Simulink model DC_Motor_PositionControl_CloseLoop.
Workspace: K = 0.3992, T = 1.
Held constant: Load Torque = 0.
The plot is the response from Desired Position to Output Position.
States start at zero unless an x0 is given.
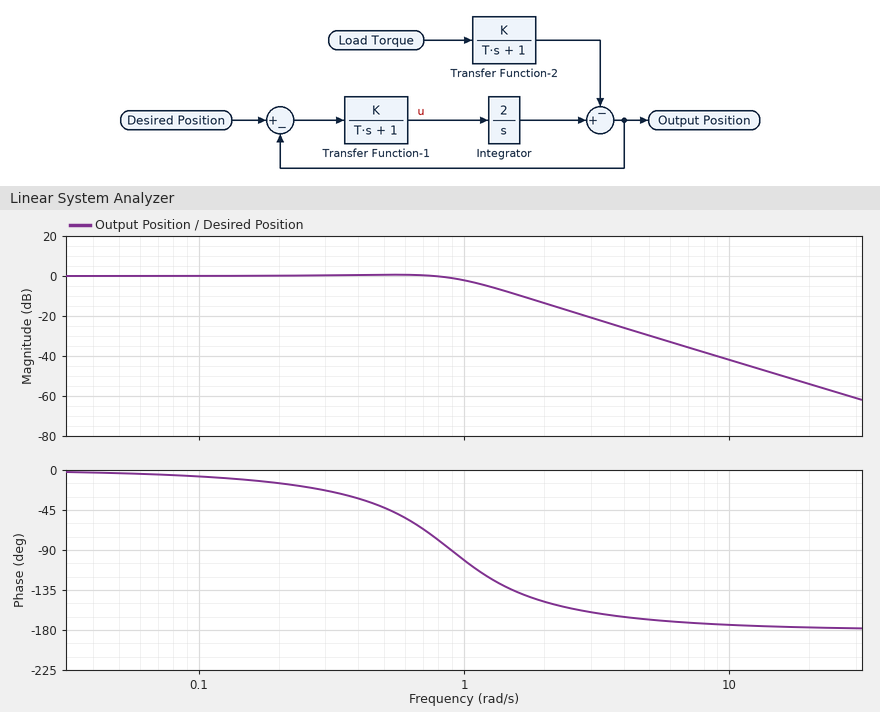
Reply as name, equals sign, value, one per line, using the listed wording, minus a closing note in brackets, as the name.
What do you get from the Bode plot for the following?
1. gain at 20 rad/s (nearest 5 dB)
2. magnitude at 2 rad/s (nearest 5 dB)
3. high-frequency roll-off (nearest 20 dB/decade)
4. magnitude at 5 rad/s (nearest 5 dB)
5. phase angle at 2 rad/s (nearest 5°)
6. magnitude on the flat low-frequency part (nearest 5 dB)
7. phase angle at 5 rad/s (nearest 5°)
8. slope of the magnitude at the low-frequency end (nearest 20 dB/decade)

gain at 20 rad/s = -55 dB
magnitude at 2 rad/s = -15 dB
high-frequency roll-off = -40 dB/decade
magnitude at 5 rad/s = -30 dB
phase angle at 2 rad/s = -150°
magnitude on the flat low-frequency part = 0 dB
phase angle at 5 rad/s = -170°
slope of the magnitude at the low-frequency end = 0 dB/decade
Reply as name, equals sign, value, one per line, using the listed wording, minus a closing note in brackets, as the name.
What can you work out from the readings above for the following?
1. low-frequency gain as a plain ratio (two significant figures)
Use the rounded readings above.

low-frequency gain as a plain ratio = 1.0
